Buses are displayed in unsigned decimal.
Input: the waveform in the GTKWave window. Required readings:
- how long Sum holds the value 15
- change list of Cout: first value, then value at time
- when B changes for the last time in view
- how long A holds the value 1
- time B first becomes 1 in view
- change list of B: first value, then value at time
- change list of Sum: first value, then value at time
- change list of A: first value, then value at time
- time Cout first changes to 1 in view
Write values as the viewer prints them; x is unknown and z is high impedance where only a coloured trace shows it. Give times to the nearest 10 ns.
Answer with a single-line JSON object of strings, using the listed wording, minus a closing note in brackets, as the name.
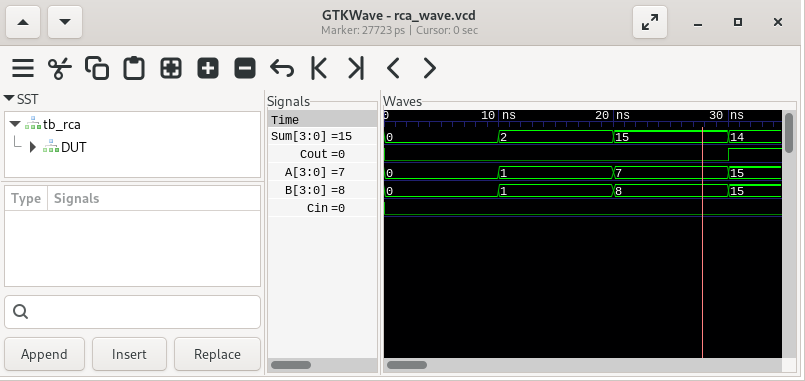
{"how long Sum holds the value 15": "10 ns", "change list of Cout: first value, then value at time": "0, 1 at 30 ns", "when B changes for the last time in view": "30 ns", "how long A holds the value 1": "10 ns", "time B first becomes 1 in view": "10 ns", "change list of B: first value, then value at time": "0, 1 at 10 ns, 8 at 20 ns, 15 at 30 ns", "change list of Sum: first value, then value at time": "0, 2 at 10 ns, 15 at 20 ns, 14 at 30 ns", "change list of A: first value, then value at time": "0, 1 at 10 ns, 7 at 20 ns, 15 at 30 ns", "time Cout first changes to 1 in view": "30 ns"}
